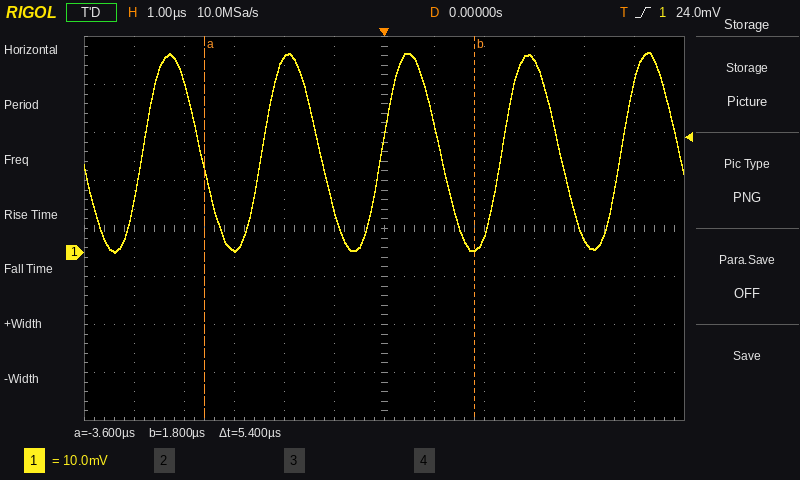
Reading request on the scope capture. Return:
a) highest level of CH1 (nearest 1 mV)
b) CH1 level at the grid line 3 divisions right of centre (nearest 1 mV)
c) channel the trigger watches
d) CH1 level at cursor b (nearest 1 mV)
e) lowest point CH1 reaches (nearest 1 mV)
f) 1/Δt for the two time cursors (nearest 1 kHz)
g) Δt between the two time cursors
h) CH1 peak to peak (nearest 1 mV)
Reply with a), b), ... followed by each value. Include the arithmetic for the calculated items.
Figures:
a) 42 mV
b) 40 mV
c) CH1
d) 1 mV
e) 0 mV
f) 1 / 5.4 µs ≈ 185 kHz
g) 5.4 µs
h) 42 mV − (0 mV) = 42 mV
